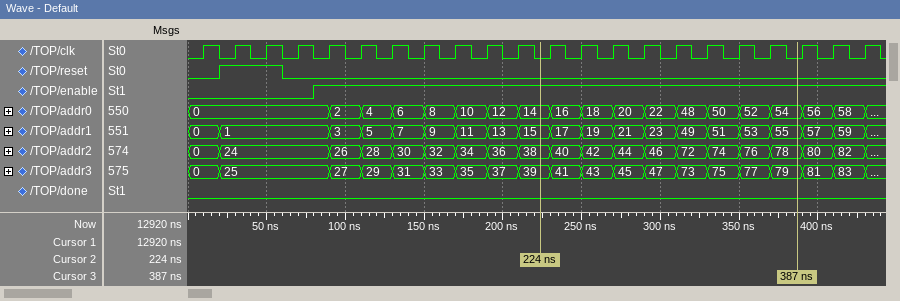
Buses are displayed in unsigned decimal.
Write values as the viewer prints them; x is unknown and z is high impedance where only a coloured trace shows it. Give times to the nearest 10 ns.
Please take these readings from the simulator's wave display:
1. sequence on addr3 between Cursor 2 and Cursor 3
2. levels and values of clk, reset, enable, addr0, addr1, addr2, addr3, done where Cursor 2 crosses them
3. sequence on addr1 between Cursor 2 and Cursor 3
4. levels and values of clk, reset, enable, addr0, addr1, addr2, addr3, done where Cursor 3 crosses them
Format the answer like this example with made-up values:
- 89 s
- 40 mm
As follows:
- 39, 41, 43, 45, 47, 73, 75, 77, 79
- clk=0, reset=0, enable=1, addr0=14, addr1=15, addr2=38, addr3=39, done=0
- 15, 17, 19, 21, 23, 49, 51, 53, 55
- clk=0, reset=0, enable=1, addr0=54, addr1=55, addr2=78, addr3=79, done=0
